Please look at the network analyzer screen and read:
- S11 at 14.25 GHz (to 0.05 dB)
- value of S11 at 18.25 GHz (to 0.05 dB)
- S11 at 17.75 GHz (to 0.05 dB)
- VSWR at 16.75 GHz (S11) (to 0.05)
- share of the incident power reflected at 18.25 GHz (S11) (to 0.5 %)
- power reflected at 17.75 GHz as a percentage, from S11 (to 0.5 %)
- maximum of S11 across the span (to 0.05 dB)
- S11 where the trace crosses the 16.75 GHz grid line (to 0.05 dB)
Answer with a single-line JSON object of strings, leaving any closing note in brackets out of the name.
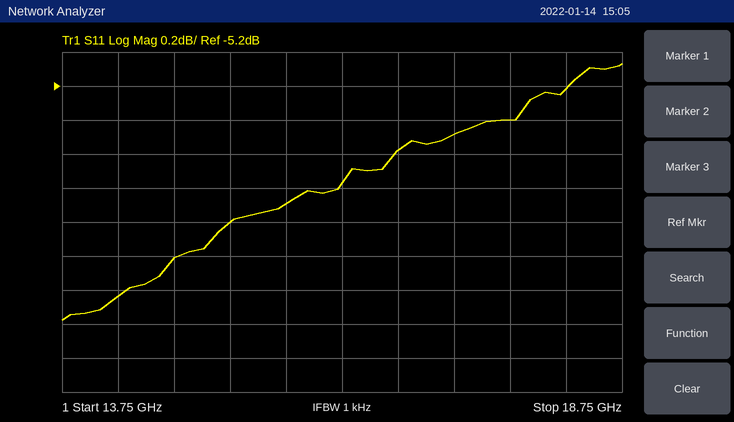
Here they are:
{"S11 at 14.25 GHz": "-6.45 dB", "value of S11 at 18.25 GHz": "-5.20 dB", "S11 at 17.75 GHz": "-5.40 dB", "VSWR at 16.75 GHz (S11)": "3.20", "share of the incident power reflected at 18.25 GHz (S11)": "30.0 %", "power reflected at 17.75 GHz as a percentage, from S11": "29.0 %", "maximum of S11 across the span": "-5.05 dB", "S11 where the trace crosses the 16.75 GHz grid line": "-5.60 dB"}
